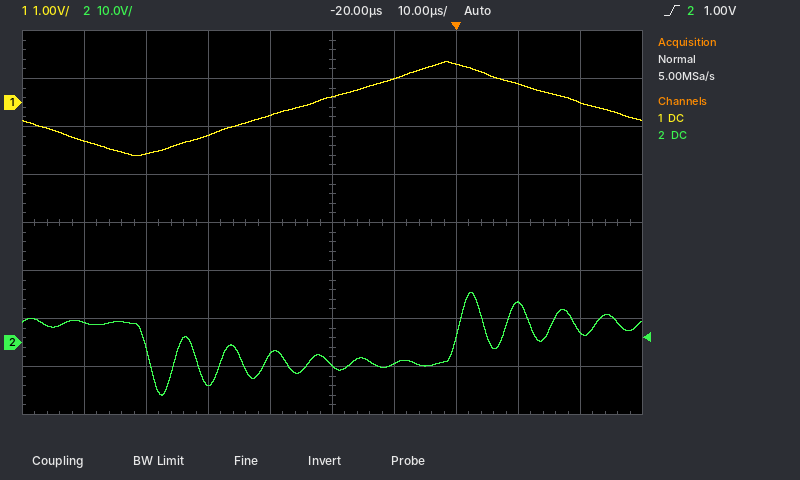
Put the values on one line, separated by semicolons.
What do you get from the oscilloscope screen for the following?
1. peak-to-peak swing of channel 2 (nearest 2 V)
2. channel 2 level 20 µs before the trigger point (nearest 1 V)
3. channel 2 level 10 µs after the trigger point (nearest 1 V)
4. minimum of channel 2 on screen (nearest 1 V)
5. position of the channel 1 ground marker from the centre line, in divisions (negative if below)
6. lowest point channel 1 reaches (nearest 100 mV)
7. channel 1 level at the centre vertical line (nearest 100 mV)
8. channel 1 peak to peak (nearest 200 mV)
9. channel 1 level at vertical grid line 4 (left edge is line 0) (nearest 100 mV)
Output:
22 V; -5 V; 8 V; -11 V; +2.5 div; -1.1 V; 100 mV; 2.0 V; -300 mV
